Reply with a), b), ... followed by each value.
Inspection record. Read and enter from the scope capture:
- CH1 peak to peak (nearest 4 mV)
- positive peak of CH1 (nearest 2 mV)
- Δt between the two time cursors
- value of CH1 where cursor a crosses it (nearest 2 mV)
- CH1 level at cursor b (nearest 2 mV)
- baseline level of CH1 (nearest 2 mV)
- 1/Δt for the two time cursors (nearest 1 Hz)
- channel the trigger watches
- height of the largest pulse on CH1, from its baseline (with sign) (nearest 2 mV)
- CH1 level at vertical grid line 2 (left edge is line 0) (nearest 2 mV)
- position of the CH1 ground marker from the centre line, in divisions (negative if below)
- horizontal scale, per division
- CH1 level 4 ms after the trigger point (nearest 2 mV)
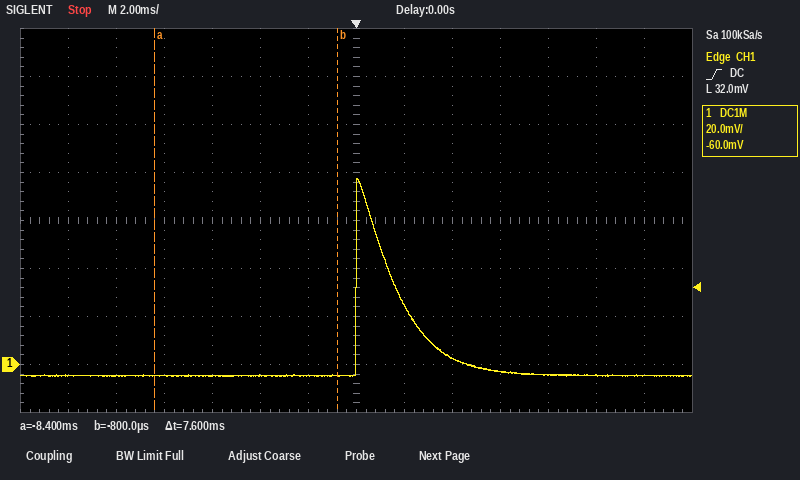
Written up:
a) 84 mV
b) 78 mV
c) 7.6 ms
d) -4 mV
e) -4 mV
f) -4 mV
g) 132 Hz
h) CH1
i) +82 mV
j) -4 mV
k) -3.0 div
l) 2 ms
m) 2 mV
